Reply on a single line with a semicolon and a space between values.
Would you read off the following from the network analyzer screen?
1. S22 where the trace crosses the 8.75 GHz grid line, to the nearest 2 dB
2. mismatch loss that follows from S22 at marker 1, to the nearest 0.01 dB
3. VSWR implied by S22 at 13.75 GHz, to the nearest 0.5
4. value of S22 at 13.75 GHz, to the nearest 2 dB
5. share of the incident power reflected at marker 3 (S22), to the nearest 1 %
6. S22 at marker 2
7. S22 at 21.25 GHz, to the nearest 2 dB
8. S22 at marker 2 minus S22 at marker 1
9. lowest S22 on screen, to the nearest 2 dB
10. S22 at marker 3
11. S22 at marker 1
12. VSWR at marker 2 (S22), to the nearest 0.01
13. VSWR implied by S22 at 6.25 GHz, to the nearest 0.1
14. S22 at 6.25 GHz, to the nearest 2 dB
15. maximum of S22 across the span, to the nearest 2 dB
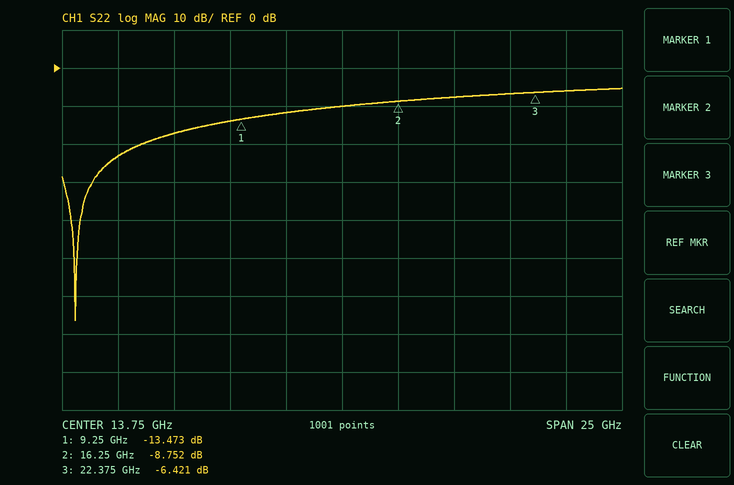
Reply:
-14 dB; 0.20 dB; 2.0; -10 dB; 23 %; -8.752 dB; -6 dB; 4.721 dB; -66 dB; -6.421 dB; -13.473 dB; 2.15; 1.3; -18 dB; -6 dB
